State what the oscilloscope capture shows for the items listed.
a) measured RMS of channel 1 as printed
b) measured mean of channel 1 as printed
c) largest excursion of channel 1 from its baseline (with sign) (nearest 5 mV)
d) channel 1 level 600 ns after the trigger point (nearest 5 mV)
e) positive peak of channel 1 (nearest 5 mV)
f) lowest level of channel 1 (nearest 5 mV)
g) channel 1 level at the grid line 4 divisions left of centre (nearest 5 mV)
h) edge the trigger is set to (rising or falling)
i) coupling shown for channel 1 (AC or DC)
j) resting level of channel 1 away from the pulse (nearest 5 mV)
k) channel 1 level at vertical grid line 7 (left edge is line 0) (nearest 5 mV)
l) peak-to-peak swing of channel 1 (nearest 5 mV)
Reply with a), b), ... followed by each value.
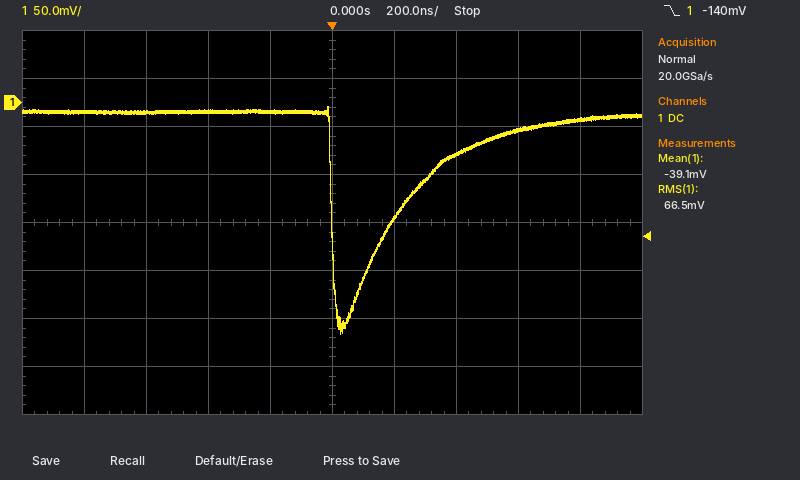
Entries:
a) 66.5 mV
b) -39.1 mV
c) -230 mV
d) -30 mV
e) -5 mV
f) -240 mV
g) -10 mV
h) falling
i) DC
j) -10 mV
k) -55 mV
l) 235 mV
